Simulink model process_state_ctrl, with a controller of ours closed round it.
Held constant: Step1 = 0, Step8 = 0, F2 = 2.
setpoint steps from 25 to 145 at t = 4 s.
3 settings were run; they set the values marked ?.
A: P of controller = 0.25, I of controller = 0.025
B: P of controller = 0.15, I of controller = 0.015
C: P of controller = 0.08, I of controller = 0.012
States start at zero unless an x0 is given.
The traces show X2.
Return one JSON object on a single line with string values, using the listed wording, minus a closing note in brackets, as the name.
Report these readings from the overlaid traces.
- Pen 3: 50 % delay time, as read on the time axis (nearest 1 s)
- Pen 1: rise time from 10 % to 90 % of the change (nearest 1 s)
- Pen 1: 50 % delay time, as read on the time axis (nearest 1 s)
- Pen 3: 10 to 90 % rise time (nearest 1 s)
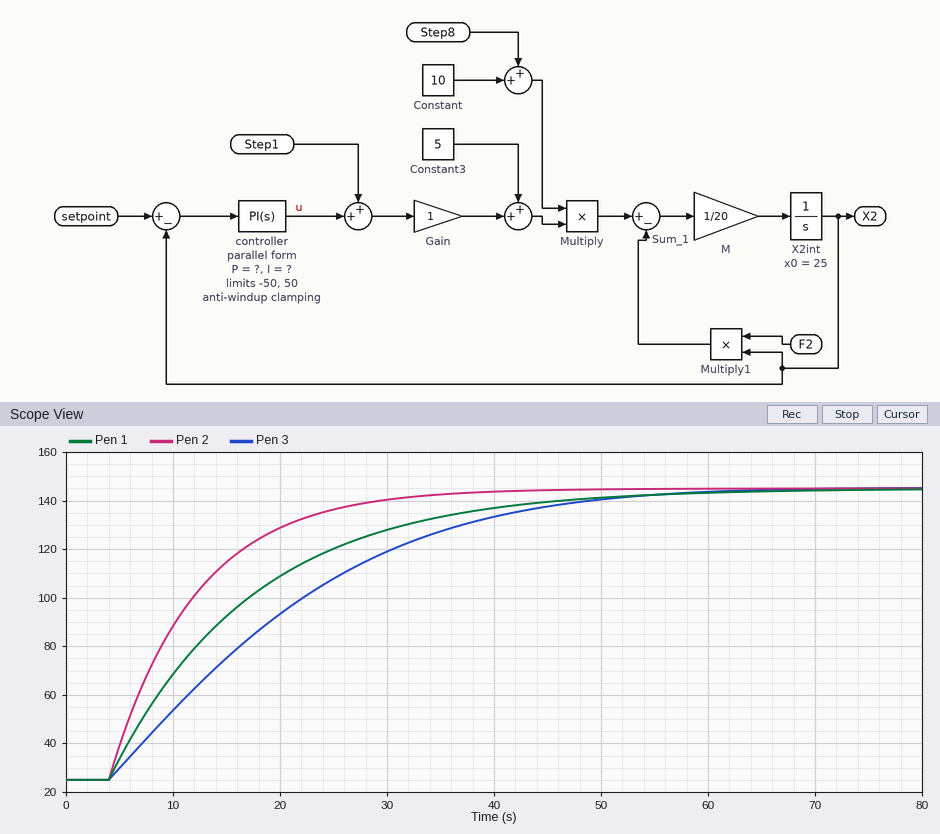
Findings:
{"Pen 3: 50 % delay time, as read on the time axis": "18 s", "Pen 1: rise time from 10 % to 90 % of the change": "29 s", "Pen 1: 50 % delay time, as read on the time axis": "13 s", "Pen 3: 10 to 90 % rise time": "33 s"}
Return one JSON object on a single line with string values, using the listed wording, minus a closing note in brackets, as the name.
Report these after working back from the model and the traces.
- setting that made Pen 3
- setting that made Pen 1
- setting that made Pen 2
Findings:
{"setting that made Pen 3": "C", "setting that made Pen 1": "B", "setting that made Pen 2": "A"}
